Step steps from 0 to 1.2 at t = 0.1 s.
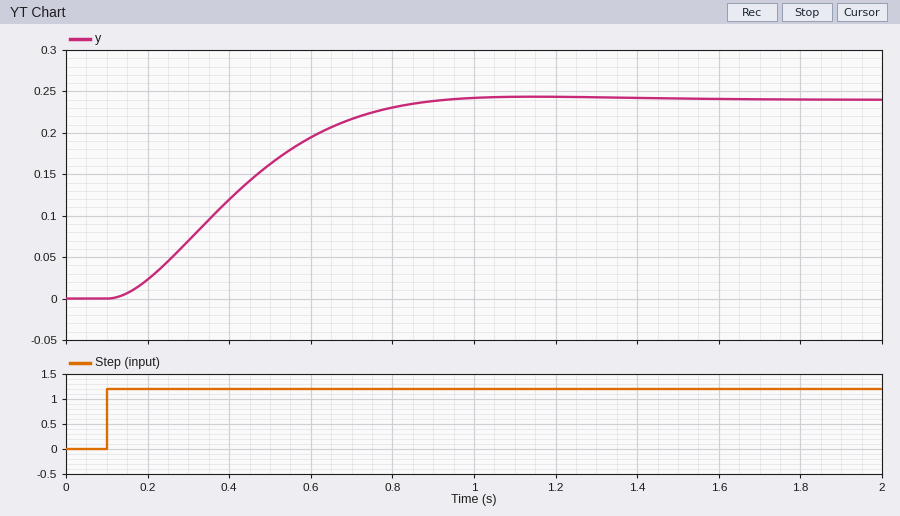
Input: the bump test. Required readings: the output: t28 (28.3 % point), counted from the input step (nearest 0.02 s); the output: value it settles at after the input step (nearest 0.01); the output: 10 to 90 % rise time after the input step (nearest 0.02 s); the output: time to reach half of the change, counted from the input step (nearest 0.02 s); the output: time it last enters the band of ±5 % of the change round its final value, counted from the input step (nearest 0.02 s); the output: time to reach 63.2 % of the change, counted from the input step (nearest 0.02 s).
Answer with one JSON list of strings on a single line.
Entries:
["0.20 s", "0.24", "0.50 s", "0.30 s", "0.68 s", "0.38 s"]
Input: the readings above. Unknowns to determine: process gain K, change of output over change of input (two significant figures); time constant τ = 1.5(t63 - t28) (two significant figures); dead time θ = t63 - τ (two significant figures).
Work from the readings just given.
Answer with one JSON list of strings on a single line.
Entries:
["0.20", "0.27 s", "0.11 s"]
